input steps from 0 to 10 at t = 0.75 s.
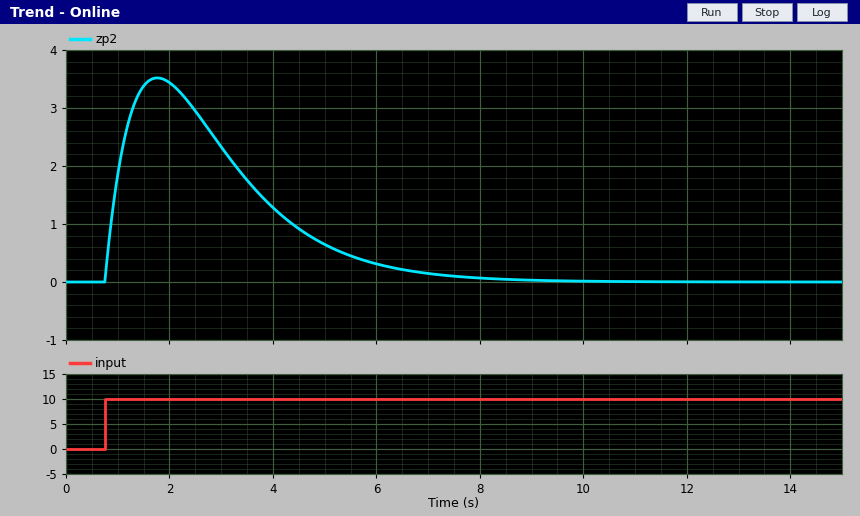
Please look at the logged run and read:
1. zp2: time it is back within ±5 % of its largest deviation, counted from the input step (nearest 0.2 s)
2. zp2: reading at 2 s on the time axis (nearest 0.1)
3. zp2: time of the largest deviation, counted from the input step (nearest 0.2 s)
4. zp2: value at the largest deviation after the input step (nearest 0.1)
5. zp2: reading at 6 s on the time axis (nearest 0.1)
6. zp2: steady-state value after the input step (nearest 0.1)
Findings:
6.0 s
3.4
1.0 s
3.5
0.3
0.0
